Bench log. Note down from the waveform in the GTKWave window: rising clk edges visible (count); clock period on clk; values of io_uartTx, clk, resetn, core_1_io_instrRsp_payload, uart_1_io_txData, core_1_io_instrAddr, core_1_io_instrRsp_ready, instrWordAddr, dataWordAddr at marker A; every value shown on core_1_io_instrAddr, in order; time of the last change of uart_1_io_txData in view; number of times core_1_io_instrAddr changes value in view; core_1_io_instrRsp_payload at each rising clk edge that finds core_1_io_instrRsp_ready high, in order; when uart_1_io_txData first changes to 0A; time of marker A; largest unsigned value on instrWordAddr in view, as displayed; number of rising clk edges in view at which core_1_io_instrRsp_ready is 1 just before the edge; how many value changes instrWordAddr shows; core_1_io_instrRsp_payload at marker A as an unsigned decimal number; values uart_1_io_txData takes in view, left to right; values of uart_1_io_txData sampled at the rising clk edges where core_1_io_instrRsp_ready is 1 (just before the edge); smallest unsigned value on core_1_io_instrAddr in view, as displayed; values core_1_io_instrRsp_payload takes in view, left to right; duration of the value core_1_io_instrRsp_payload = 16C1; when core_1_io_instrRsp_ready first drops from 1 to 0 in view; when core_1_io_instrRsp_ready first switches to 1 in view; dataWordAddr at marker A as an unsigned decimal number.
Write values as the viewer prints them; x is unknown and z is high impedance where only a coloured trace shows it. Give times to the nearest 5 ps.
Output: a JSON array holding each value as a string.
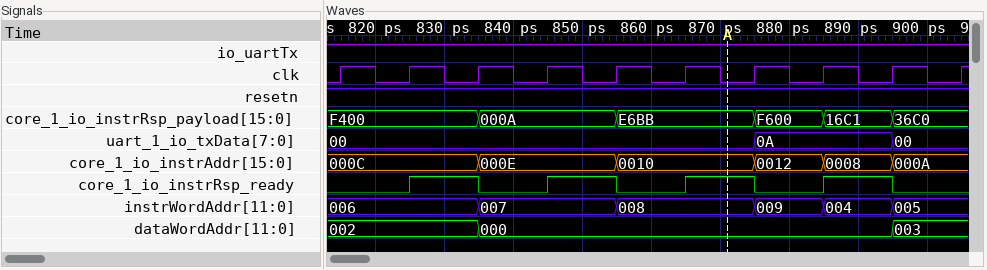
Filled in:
["10", "10 ps", "io_uartTx=1, clk=0, resetn=1, core_1_io_instrRsp_payload=E6BB, uart_1_io_txData=00, core_1_io_instrAddr=0010, core_1_io_instrRsp_ready=1, instrWordAddr=008, dataWordAddr=000", "000C, 000E, 0010, 0012, 0008, 000A", "895 ps", "5", "F400, 000A, E6BB, 16C1", "875 ps", "870 ps", "009", "4", "5", "59067", "00, 0A, 00", "00, 00, 00, 0A", "0008", "F400, 000A, E6BB, F600, 16C1, 36C0", "10 ps", "835 ps", "825 ps", "0"]
